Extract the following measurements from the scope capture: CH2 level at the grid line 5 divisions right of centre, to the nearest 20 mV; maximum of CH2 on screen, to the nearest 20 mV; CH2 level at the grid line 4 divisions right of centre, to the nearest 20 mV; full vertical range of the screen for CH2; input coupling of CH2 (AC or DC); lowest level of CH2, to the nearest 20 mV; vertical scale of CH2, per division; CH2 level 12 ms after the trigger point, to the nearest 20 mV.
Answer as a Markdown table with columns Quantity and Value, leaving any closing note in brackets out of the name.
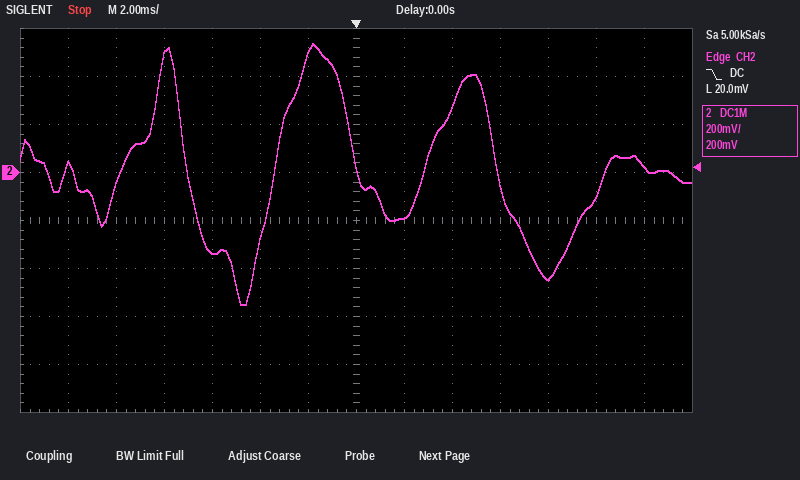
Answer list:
| Quantity | Value |
|---|---|
| CH2 level at the grid line 5 divisions right of centre, to the nearest 20 mV | -100 mV |
| maximum of CH2 on screen, to the nearest 20 mV | 540 mV |
| CH2 level at the grid line 4 divisions right of centre, to the nearest 20 mV | -440 mV |
| full vertical range of the screen for CH2 | 1.6 V |
| input coupling of CH2 | DC |
| lowest level of CH2, to the nearest 20 mV | -560 mV |
| vertical scale of CH2, per division | 200 mV |
| CH2 level 12 ms after the trigger point, to the nearest 20 mV | 20 mV |
